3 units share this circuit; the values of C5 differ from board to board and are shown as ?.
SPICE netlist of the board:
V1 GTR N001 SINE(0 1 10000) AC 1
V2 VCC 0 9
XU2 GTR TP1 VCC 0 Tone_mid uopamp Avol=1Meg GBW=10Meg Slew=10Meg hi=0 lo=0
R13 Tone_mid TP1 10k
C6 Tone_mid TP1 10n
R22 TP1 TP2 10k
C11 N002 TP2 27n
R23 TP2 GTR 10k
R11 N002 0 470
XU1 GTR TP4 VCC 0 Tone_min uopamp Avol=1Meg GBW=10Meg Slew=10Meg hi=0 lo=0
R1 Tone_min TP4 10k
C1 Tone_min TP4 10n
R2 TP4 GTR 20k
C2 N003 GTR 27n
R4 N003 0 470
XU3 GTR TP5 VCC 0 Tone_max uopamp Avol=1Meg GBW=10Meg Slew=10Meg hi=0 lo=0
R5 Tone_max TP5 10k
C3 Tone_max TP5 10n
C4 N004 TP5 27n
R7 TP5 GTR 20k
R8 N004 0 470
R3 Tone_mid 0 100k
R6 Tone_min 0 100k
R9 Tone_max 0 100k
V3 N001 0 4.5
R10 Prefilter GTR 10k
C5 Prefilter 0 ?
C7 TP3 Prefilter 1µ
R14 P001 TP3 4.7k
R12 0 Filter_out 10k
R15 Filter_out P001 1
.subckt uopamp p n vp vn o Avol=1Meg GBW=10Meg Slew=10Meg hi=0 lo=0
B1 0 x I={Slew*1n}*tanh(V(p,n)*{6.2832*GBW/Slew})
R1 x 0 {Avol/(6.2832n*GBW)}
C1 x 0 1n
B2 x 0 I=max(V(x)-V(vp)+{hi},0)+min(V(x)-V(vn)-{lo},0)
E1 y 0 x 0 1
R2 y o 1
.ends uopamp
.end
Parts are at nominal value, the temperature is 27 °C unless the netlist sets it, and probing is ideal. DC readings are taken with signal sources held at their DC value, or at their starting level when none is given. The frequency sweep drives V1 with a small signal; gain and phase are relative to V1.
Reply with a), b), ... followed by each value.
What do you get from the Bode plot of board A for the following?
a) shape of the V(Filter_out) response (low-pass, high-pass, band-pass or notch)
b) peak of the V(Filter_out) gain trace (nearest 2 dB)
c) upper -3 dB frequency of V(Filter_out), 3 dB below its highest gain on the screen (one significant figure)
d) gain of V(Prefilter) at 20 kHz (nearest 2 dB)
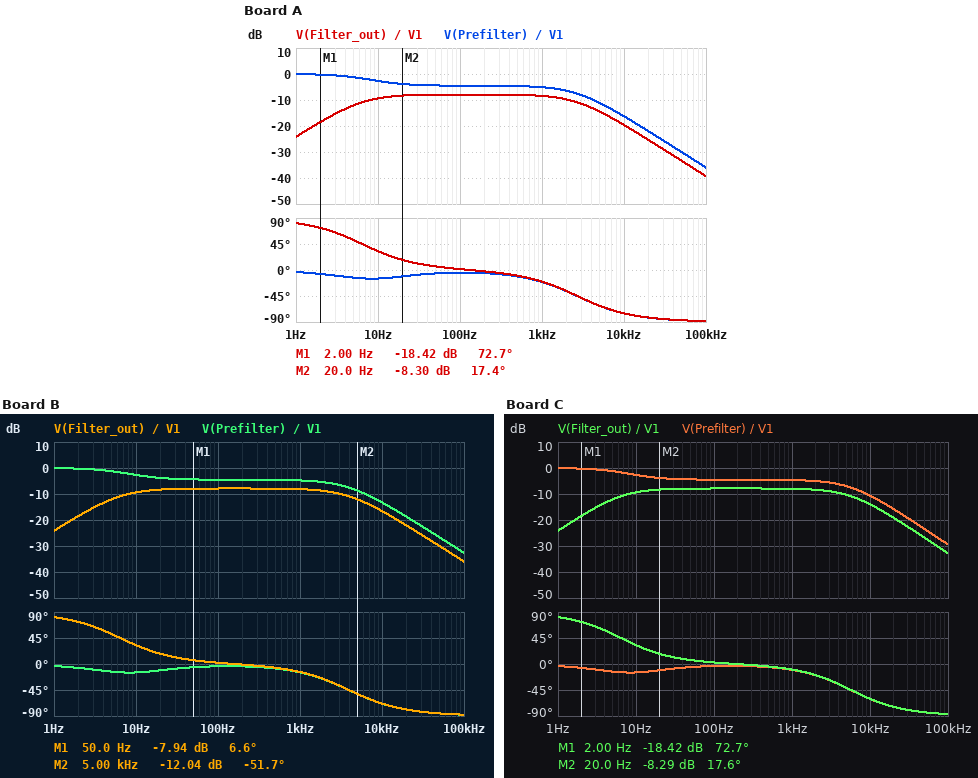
a) band-pass
b) -8 dB
c) 3 kHz
d) -22 dB
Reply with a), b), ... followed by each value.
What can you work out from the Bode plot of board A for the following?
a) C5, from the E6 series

a) 10 nF
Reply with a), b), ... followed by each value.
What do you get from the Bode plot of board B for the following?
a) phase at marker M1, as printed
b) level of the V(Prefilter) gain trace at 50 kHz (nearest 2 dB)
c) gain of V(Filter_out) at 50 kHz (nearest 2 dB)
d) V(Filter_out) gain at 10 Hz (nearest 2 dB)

a) 6.6 deg
b) -26 dB
c) -30 dB
d) -10 dB
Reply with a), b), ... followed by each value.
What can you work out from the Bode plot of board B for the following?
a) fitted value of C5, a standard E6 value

a) 6.8 nF
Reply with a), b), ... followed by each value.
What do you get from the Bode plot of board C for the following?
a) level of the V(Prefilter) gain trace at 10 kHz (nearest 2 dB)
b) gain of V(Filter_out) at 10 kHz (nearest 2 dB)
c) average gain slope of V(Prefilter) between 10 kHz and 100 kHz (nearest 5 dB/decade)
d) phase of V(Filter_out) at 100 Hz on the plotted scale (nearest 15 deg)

a) -10 dB
b) -14 dB
c) -20 dB/decade
d) 0 deg
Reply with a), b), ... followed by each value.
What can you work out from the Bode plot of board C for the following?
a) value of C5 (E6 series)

a) 4.7 nF
